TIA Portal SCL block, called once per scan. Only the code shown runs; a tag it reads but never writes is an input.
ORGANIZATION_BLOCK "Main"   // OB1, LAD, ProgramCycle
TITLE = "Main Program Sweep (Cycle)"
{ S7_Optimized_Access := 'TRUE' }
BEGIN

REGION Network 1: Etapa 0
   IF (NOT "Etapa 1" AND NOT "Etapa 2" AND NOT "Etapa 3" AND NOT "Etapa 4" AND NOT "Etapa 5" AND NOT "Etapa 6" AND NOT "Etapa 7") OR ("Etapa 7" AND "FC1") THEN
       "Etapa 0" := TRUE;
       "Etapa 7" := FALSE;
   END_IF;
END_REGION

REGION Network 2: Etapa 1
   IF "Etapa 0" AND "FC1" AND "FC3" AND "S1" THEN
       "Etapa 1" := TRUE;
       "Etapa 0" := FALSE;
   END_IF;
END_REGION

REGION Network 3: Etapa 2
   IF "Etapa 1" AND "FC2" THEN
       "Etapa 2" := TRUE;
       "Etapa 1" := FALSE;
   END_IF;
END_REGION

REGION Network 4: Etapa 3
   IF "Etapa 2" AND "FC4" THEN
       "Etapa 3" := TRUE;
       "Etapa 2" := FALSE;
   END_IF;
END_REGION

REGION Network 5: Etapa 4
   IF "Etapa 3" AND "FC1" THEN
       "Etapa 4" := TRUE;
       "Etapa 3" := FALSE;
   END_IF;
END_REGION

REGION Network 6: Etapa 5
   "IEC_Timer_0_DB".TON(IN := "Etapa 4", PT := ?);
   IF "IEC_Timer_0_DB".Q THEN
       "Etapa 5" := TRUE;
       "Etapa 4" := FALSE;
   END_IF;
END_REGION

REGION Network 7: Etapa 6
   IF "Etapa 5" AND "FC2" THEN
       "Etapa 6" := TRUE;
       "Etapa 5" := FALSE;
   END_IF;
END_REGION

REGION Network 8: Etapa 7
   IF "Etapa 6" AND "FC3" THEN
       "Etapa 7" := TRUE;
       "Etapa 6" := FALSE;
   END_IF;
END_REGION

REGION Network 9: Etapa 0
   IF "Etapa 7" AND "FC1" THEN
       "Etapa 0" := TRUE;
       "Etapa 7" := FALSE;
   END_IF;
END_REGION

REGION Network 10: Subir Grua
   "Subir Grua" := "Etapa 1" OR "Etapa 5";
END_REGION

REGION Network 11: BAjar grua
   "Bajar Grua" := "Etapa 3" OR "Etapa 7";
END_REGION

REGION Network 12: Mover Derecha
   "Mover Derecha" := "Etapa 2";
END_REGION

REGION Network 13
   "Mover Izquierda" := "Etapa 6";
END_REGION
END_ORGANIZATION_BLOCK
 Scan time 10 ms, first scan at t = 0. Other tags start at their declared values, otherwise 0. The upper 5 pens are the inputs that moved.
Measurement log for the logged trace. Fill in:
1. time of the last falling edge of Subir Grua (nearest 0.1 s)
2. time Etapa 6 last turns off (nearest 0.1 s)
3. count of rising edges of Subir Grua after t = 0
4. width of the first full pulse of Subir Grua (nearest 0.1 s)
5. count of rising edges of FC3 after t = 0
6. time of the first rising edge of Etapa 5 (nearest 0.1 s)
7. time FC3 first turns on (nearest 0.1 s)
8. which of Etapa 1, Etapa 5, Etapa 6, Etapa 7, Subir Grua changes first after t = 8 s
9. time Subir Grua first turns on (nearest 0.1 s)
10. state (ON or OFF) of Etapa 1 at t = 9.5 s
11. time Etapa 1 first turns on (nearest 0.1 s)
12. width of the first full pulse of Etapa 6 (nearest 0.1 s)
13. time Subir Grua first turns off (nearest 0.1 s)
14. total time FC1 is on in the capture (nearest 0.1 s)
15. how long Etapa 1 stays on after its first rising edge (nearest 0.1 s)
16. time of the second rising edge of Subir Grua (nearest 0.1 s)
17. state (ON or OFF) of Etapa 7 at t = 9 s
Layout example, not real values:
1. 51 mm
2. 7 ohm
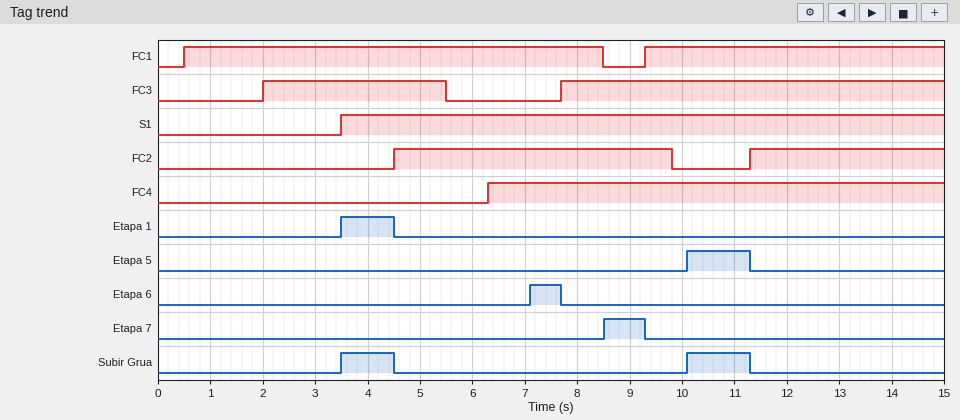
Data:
1. 11.3 s
2. 7.7 s
3. 2
4. 1.0 s
5. 2
6. 10.1 s
7. 2.0 s
8. Etapa 7
9. 3.5 s
10. OFF
11. 3.5 s
12. 0.6 s
13. 4.5 s
14. 13.7 s
15. 1.0 s
16. 10.1 s
17. ON
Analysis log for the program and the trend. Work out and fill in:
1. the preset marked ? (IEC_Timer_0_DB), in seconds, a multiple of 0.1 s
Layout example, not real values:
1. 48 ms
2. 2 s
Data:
1. 0.8 s
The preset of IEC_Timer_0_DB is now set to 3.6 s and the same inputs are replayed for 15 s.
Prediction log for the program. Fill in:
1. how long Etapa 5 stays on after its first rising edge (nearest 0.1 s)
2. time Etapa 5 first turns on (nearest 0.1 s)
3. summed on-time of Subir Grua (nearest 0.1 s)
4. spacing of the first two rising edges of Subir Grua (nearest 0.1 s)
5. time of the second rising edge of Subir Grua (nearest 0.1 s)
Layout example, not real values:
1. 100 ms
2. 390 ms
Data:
1. 1.4 s
2. 9.9 s
3. 2.4 s
4. 6.4 s
5. 9.9 s
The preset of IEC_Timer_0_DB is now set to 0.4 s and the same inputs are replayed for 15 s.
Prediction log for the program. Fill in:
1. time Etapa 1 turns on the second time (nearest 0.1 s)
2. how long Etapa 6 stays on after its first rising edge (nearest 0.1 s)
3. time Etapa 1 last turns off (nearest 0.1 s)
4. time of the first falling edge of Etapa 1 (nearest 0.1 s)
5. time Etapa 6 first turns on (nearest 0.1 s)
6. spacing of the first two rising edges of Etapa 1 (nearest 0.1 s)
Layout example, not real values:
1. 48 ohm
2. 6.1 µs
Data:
1. 9.8 s
2. 1.0 s
3. 11.3 s
4. 4.5 s
5. 6.7 s
6. 6.3 s
